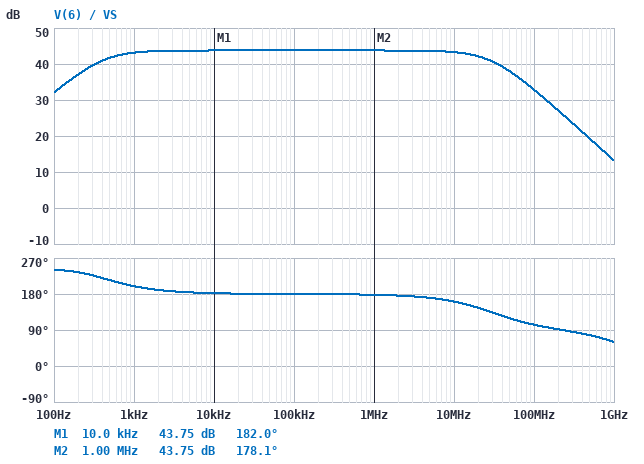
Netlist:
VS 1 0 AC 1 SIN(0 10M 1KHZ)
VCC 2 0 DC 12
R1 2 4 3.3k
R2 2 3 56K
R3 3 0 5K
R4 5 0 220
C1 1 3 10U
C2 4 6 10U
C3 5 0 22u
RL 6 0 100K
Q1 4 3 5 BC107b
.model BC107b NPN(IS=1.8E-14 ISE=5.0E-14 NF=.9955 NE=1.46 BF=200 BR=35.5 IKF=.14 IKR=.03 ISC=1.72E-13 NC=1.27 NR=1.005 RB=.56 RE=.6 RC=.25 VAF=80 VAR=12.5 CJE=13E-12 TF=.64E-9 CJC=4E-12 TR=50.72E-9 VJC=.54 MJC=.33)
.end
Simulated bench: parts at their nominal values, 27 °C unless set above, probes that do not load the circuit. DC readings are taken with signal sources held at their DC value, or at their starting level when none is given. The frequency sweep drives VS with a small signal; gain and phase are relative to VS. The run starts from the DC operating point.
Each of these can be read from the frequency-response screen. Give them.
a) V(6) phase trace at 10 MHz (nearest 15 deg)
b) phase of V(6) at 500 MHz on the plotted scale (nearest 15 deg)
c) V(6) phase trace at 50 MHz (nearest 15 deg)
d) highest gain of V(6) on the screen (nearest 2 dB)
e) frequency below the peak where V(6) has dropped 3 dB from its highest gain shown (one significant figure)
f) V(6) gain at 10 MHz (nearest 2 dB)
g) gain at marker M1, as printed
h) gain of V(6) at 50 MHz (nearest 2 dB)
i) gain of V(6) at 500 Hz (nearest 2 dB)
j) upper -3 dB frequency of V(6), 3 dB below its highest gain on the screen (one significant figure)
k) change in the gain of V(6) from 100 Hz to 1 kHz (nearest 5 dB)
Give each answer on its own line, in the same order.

165 deg
75 deg
120 deg
44 dB
400 Hz
44 dB
43.75 dB
38 dB
42 dB
30 MHz
10 dB
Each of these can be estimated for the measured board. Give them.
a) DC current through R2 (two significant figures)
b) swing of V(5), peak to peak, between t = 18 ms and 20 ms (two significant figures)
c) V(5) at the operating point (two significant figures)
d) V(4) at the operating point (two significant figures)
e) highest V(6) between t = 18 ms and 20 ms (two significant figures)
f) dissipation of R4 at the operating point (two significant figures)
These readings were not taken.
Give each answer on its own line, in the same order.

200 µA
6.5 mV
300 mV
7.5 V
1.3 V
410 µW
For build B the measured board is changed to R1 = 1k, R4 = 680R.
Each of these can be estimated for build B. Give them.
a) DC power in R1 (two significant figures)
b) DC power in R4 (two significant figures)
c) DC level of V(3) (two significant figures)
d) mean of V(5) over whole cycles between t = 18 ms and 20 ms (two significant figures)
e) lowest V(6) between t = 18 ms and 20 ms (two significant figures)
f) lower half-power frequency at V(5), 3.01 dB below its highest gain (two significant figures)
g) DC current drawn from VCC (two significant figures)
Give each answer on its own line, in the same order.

260 µW
180 µW
970 mV
350 mV
-210 mV
3.4 Hz
710 µA
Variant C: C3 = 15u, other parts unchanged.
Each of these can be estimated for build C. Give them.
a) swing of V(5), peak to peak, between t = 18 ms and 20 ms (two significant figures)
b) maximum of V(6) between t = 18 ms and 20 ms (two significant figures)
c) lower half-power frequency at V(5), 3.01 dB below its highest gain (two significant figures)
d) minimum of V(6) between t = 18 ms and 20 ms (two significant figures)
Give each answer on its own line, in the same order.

8.9 mV
1.2 V
3.8 Hz
-1.4 V
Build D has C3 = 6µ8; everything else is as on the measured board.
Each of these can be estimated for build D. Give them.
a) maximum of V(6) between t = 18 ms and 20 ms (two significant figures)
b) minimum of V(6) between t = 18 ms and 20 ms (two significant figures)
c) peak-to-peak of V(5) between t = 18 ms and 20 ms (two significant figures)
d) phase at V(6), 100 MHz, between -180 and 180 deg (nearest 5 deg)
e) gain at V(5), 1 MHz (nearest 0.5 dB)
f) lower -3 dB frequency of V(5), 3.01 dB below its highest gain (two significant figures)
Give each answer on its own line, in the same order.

930 mV
-1.0 V
14 mV
105 deg
-59.0 dB
3.8 Hz
